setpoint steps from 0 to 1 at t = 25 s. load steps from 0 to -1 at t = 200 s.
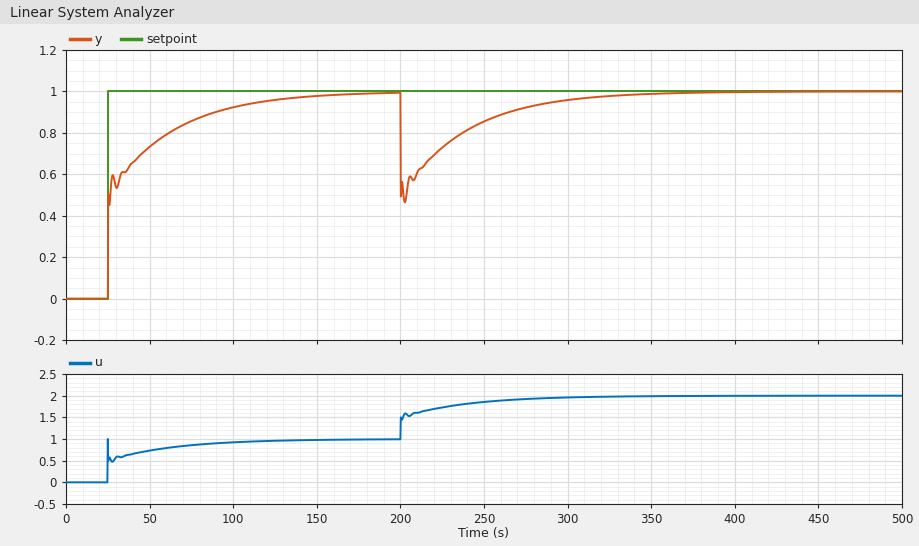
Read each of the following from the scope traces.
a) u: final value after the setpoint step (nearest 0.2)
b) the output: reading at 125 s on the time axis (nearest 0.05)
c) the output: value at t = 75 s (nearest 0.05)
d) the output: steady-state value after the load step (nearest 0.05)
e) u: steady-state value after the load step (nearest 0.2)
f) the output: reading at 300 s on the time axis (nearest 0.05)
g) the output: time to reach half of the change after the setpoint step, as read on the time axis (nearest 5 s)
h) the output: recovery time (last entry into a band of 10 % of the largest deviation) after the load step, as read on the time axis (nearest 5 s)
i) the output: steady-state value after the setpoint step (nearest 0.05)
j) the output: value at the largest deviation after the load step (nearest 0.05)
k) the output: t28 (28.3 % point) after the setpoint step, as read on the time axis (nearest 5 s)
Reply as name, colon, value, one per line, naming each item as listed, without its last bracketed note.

u: final value after the setpoint step: 1.0
the output: reading at 125 s on the time axis: 0.95
the output: value at t = 75 s: 0.85
the output: steady-state value after the load step: 1.00
u: steady-state value after the load step: 2.0
the output: reading at 300 s on the time axis: 0.95
the output: time to reach half of the change after the setpoint step, as read on the time axis: 25 s
the output: recovery time (last entry into a band of 10 % of the largest deviation) after the load step, as read on the time axis: 290 s
the output: steady-state value after the setpoint step: 1.00
the output: value at the largest deviation after the load step: 0.45
the output: t28 (28.3 % point) after the setpoint step, as read on the time axis: 25 s
